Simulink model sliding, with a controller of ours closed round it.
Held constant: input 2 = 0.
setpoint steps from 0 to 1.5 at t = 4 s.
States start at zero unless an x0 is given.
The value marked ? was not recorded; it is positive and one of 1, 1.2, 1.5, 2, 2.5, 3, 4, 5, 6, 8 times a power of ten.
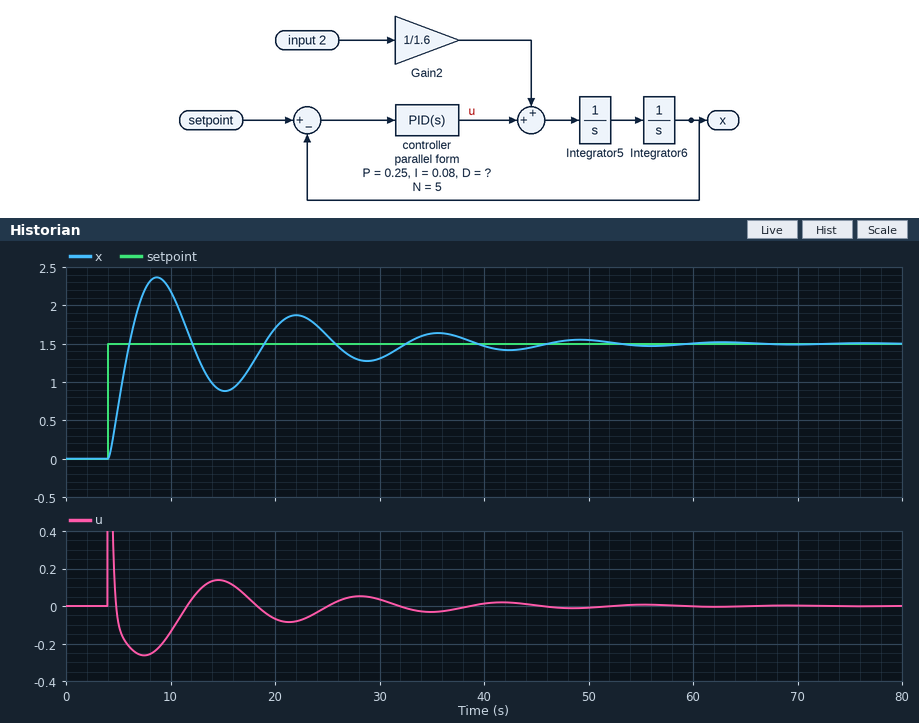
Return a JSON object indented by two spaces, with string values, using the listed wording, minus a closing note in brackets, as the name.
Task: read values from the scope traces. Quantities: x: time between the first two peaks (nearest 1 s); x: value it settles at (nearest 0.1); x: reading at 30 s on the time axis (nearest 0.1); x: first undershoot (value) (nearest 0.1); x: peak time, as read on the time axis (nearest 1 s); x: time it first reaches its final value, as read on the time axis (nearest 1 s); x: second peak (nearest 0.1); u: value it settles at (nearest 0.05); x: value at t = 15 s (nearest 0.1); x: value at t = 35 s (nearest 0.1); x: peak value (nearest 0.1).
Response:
{
  "x: time between the first two peaks": "13 s",
  "x: value it settles at": "1.5",
  "x: reading at 30 s on the time axis": "1.3",
  "x: first undershoot (value)": "0.9",
  "x: peak time, as read on the time axis": "9 s",
  "x: time it first reaches its final value, as read on the time axis": "6 s",
  "x: second peak": "1.9",
  "u: value it settles at": "0.00",
  "x: value at t = 15 s": "0.9",
  "x: value at t = 35 s": "1.6",
  "x: peak value": "2.4"
}
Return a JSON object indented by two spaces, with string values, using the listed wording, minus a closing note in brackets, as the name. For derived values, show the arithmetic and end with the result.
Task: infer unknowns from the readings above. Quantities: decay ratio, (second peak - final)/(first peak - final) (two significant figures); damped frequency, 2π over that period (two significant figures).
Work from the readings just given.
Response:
{
  "decay ratio, (second peak - final)/(first peak - final)": "(1.9 - 1.5) / (2.4 - 1.5) = 0.44",
  "damped frequency, 2π over that period": "2π / 13 = 0.48 rad/s"
}
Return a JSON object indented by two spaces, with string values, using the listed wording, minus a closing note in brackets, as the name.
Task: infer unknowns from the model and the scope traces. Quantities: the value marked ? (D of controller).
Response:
{
  "the value marked ?": "0.5"
}
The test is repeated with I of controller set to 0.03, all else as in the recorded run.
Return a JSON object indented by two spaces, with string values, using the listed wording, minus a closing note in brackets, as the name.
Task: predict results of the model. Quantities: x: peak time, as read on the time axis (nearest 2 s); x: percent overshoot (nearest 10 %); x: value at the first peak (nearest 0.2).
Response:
{
  "x: peak time, as read on the time axis": "8 s",
  "x: percent overshoot": "40 %",
  "x: value at the first peak": "2.2"
}
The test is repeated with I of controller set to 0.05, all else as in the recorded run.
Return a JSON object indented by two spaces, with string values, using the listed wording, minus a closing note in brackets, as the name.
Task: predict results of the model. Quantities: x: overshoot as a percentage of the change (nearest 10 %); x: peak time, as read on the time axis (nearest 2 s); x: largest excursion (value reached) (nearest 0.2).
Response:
{
  "x: overshoot as a percentage of the change": "50 %",
  "x: peak time, as read on the time axis": "8 s",
  "x: largest excursion (value reached)": "2.2"
}
